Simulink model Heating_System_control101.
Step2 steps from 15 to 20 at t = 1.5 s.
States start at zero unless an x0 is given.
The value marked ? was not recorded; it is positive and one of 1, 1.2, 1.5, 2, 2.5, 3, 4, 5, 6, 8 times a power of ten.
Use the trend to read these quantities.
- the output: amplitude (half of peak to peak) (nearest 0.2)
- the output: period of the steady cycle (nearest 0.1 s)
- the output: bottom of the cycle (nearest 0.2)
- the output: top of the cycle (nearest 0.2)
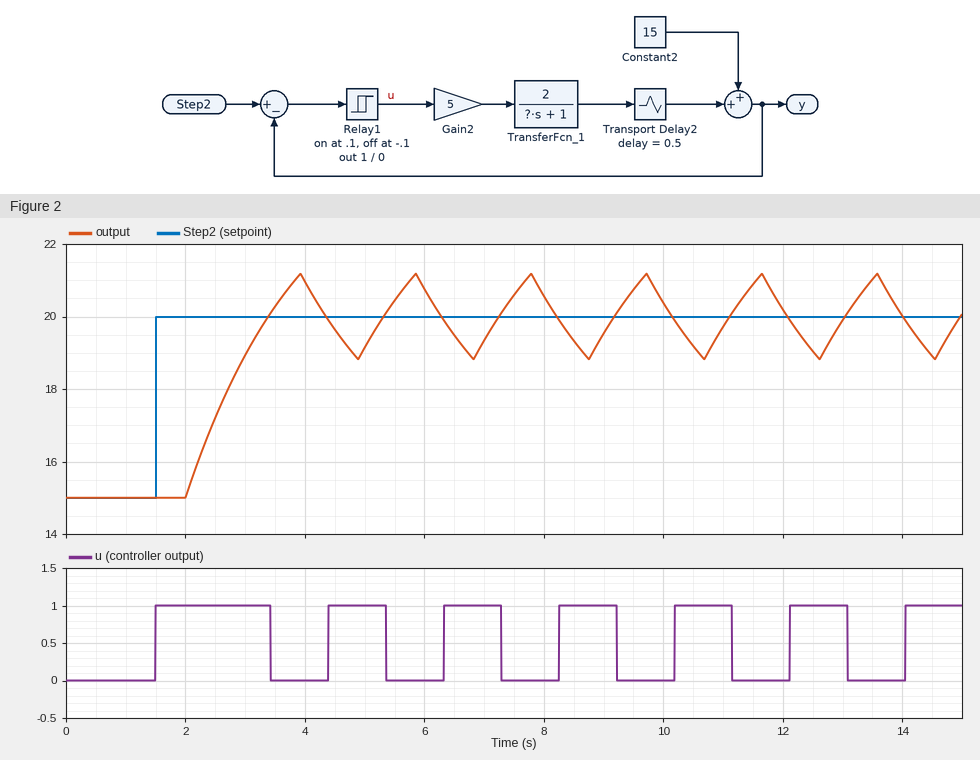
1.2
1.9 s
18.8
21.2
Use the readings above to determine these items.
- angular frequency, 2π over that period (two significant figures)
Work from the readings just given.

3.3 rad/s
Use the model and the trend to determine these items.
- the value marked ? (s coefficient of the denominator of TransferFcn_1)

2
